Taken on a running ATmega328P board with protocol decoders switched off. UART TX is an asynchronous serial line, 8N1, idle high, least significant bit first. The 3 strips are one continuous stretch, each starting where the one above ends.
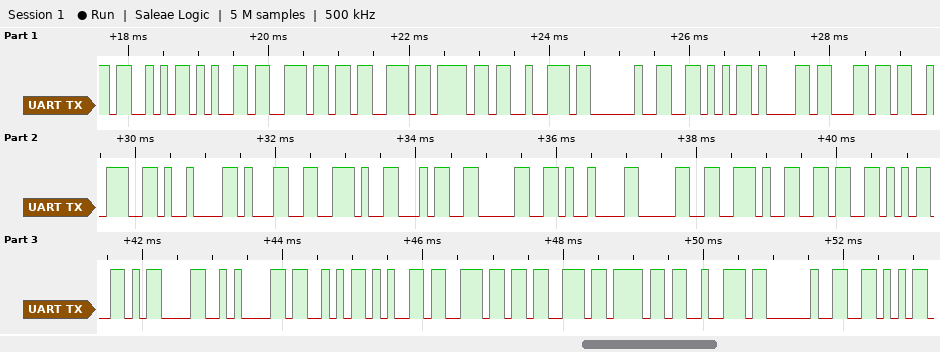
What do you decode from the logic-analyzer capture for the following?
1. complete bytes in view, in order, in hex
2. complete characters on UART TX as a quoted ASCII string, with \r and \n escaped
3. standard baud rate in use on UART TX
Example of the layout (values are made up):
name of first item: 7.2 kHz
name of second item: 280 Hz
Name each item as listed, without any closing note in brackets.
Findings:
complete bytes in view, in order, in hex: 53 65 6E 73 6F 72 20 56 61 6C 3A 09 31 2E 34 30 09 30 2E 36 35 0D 0A 53 65 6E 73 6F 72 20 56
complete characters on UART TX as a quoted ASCII string, with \r and \n escaped: "Sensor Val:\t1.40\t0.65\r\nSensor V"
standard baud rate in use on UART TX: 9600 baud
